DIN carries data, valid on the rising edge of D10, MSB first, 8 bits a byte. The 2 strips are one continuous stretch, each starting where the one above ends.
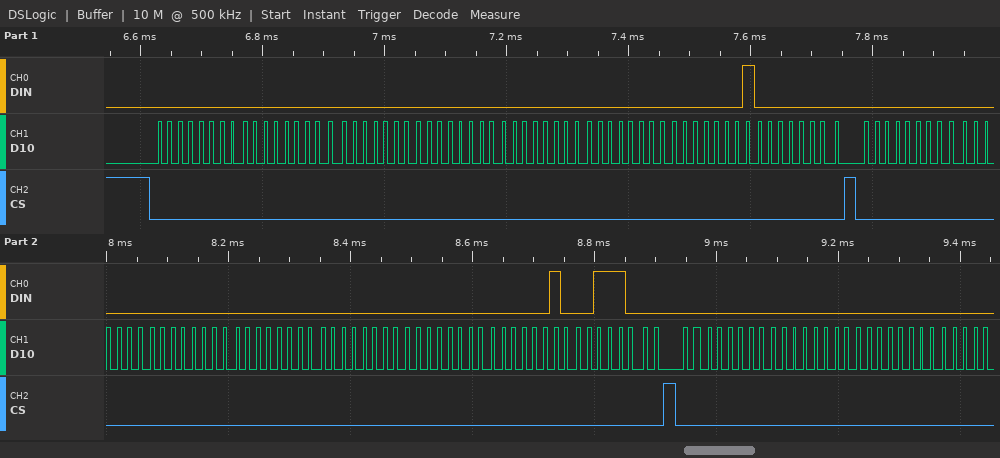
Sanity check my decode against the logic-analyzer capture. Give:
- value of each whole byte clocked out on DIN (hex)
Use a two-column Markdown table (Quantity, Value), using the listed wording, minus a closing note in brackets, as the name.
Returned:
| Quantity | Value |
|---|---|
| value of each whole byte clocked out on DIN | 00 00 00 00 00 00 01 00 00 00 00 00 00 00 02 38 00 00 00 |
